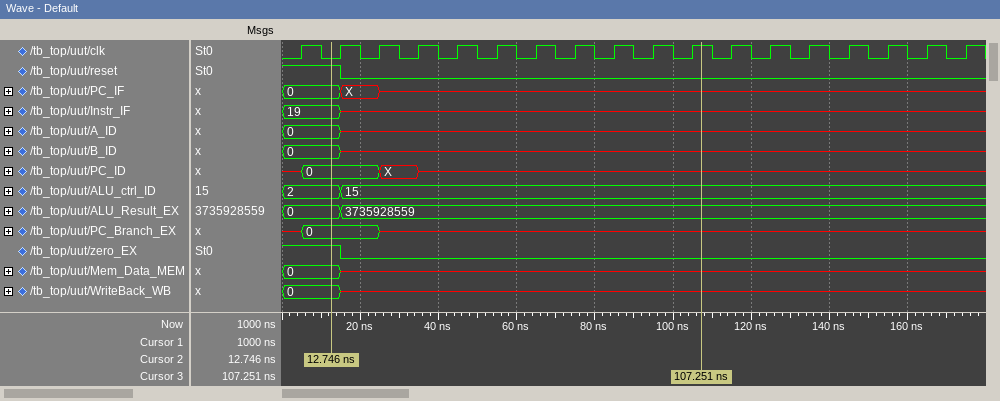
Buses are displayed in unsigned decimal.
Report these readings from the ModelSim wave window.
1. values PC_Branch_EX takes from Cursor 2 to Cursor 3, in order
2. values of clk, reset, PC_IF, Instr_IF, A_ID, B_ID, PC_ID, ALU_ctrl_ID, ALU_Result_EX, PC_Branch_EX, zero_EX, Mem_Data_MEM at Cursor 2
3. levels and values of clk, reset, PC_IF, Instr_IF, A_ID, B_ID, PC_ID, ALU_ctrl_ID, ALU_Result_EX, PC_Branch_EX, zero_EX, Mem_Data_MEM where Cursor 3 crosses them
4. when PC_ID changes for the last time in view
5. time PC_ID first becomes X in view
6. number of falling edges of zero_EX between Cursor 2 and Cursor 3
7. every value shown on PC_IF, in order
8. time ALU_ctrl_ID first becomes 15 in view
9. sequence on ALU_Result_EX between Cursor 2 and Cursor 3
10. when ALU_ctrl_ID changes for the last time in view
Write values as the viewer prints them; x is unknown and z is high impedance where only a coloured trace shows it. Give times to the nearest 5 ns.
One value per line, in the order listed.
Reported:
0, x
clk=0, reset=1, PC_IF=0, Instr_IF=19, A_ID=0, B_ID=0, PC_ID=0, ALU_ctrl_ID=2, ALU_Result_EX=0, PC_Branch_EX=0, zero_EX=1, Mem_Data_MEM=0
clk=1, reset=0, PC_IF=x, Instr_IF=x, A_ID=x, B_ID=x, PC_ID=x, ALU_ctrl_ID=15, ALU_Result_EX=3735928559, PC_Branch_EX=x, zero_EX=0, Mem_Data_MEM=x
35 ns
25 ns
1
0, X, x
15 ns
0, 3735928559
15 ns
